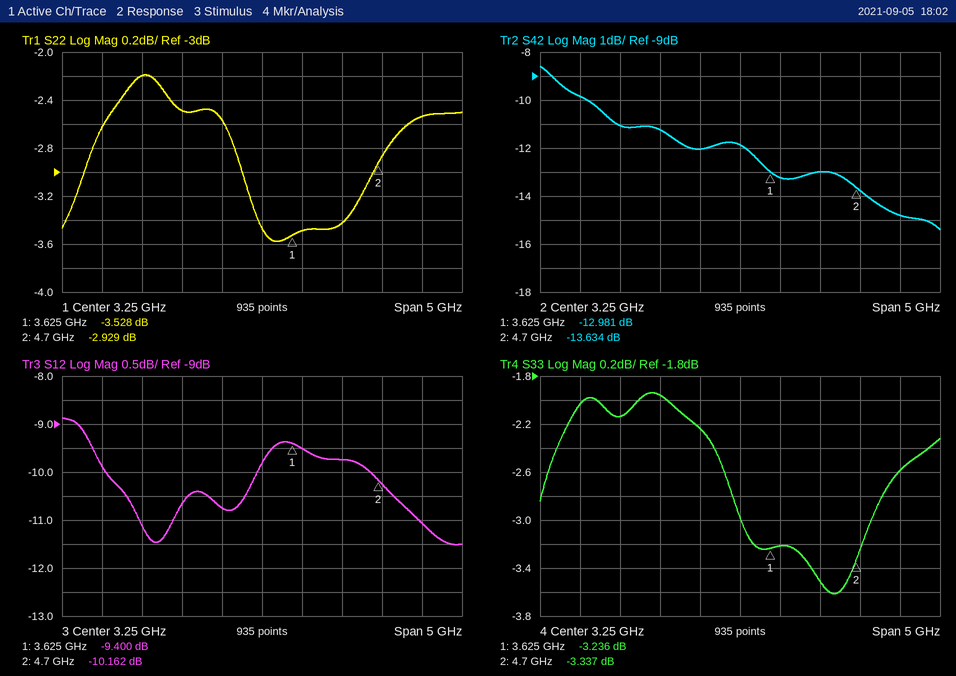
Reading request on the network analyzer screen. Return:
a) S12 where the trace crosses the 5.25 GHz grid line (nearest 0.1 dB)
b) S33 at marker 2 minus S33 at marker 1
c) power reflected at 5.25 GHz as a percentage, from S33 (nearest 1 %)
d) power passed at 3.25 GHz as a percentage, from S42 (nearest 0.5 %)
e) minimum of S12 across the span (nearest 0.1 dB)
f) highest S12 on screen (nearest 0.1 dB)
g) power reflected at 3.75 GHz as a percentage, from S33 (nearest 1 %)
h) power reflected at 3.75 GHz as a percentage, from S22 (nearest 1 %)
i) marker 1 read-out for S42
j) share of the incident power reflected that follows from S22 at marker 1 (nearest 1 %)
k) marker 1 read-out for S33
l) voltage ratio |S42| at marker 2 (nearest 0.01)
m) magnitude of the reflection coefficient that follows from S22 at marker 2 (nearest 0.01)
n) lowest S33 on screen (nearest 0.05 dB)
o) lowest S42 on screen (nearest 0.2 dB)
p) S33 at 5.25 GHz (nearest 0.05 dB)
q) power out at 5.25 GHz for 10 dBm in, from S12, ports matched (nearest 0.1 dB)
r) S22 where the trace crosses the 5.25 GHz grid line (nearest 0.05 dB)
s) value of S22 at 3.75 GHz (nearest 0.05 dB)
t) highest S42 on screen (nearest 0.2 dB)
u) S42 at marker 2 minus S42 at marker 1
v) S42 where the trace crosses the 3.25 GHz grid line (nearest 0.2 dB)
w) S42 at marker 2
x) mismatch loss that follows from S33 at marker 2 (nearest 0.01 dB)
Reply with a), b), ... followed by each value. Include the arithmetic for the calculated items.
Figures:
a) -11.1 dB
b) -3.337 − (-3.236) = -0.101 dB
c) 10^(-2.6/10) ≈ 55 %
d) 10^(-11.8/10) ≈ 6.61 %, so 6.5 % to the nearest 0.5 %
e) -11.5 dB
f) -8.9 dB
g) 10^(-3.2/10) ≈ 48 %
h) 10^(-3.5/10) ≈ 45 %
i) -12.981 dB
j) 10^(-3.528/10) ≈ 44 %
k) -3.236 dB
l) 10^(-13.634/20) ≈ 0.21
m) 10^(-2.929/20) ≈ 0.71
n) -3.60 dB
o) -15.4 dB
p) -2.60 dB
q) 10 dBm + (-11.1 dB) = -1.1 dBm
r) -2.55 dB
s) -3.50 dB
t) -8.6 dB
u) -13.634 − (-12.981) = -0.653 dB
v) -11.8 dB
w) -13.634 dB
x) −10 log10(1 − 10^(-3.337/10)) ≈ 2.71 dB
